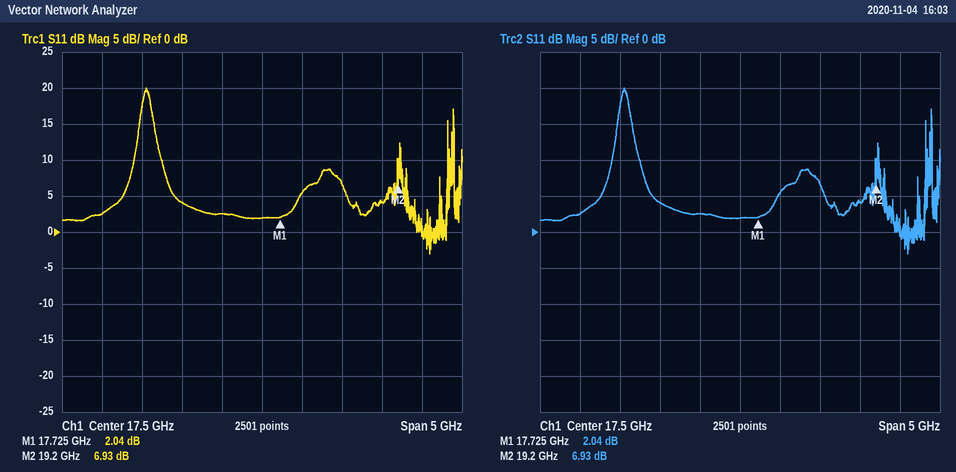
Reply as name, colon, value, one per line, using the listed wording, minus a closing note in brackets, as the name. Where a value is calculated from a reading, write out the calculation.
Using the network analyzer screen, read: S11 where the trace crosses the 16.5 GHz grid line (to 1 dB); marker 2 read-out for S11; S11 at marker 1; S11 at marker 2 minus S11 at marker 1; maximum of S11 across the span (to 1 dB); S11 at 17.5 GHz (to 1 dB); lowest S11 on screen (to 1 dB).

S11 where the trace crosses the 16.5 GHz grid line: 4 dB
marker 2 read-out for S11: 6.93 dB
S11 at marker 1: 2.04 dB
S11 at marker 2 minus S11 at marker 1: 6.93 − (2.04) = 4.89 dB
maximum of S11 across the span: 20 dB
S11 at 17.5 GHz: 2 dB
lowest S11 on screen: -3 dB
